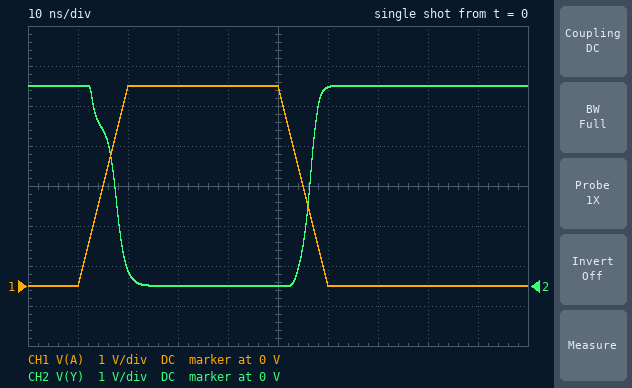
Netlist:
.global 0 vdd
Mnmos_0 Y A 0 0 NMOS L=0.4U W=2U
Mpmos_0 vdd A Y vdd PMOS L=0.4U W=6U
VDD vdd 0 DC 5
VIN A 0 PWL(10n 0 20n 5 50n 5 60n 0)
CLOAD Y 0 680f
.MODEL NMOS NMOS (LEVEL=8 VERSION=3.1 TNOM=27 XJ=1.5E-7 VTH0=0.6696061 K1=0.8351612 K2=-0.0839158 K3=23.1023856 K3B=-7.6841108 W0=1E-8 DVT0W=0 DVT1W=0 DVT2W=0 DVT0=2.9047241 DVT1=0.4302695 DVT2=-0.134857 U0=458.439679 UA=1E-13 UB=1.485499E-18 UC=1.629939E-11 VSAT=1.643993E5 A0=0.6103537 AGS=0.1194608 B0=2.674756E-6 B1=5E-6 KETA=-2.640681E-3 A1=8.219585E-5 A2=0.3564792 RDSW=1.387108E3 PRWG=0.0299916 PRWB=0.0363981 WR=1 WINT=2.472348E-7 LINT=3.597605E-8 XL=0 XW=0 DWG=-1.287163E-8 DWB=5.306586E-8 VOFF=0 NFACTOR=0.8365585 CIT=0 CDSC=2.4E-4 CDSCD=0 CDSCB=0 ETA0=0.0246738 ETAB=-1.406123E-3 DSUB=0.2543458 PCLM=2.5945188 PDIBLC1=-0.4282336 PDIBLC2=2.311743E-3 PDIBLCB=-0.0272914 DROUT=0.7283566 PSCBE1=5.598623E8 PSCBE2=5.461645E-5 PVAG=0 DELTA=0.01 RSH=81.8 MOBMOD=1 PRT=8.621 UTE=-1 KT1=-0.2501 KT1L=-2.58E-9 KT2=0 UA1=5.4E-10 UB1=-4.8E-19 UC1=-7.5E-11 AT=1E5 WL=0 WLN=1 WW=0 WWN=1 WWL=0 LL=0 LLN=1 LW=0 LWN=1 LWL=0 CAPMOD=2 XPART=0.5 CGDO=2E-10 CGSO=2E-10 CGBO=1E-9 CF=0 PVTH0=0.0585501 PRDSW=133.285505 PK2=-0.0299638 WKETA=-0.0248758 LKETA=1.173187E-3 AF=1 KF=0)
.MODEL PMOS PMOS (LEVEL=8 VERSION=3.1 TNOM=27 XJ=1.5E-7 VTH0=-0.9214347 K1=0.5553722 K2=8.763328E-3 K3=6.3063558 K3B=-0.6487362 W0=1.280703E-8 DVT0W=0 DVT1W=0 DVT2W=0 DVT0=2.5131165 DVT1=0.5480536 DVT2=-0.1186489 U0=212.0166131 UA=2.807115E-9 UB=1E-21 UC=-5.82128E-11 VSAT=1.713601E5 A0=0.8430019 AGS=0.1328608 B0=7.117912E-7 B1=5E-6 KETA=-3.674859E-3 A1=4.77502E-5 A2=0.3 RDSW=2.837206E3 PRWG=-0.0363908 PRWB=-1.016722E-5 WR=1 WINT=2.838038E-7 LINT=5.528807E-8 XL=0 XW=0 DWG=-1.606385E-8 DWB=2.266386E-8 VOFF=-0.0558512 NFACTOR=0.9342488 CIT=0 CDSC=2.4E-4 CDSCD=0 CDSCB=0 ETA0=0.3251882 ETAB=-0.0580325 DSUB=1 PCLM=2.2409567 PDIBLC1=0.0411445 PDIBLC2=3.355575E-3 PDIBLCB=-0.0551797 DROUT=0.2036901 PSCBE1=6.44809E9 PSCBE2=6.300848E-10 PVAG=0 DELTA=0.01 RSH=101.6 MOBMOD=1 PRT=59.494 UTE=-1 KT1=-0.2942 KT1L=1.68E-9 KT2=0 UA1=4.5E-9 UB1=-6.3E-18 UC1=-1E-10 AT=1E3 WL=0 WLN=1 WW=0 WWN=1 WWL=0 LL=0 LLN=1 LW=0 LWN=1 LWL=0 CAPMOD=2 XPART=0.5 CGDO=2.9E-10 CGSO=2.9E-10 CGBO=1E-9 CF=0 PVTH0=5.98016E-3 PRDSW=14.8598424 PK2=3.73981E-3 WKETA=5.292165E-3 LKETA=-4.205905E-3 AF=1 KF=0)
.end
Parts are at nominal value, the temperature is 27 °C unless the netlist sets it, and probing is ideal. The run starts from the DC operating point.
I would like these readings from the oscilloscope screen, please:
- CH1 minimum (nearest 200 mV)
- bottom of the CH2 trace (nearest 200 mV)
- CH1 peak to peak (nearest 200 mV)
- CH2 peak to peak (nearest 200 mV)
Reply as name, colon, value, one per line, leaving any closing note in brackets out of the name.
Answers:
CH1 minimum: 0 V
bottom of the CH2 trace: 0 V
CH1 peak to peak: 5.0 V
CH2 peak to peak: 5.0 V
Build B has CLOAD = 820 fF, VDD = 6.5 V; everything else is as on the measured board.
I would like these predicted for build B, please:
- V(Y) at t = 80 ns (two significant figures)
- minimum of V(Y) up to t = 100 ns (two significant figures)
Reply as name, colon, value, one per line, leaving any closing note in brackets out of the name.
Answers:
V(Y) at t = 80 ns: 6.5 V
minimum of V(Y) up to t = 100 ns: 360 mV
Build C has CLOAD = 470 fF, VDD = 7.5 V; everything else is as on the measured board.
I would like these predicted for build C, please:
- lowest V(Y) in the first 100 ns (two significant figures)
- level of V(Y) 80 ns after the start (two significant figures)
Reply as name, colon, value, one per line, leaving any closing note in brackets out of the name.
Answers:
lowest V(Y) in the first 100 ns: 2.0 V
level of V(Y) 80 ns after the start: 7.5 V
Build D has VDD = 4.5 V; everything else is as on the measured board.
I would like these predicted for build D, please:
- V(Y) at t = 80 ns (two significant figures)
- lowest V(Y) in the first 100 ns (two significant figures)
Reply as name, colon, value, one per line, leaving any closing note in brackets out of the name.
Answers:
V(Y) at t = 80 ns: 4.5 V
lowest V(Y) in the first 100 ns: -3.7 mV
